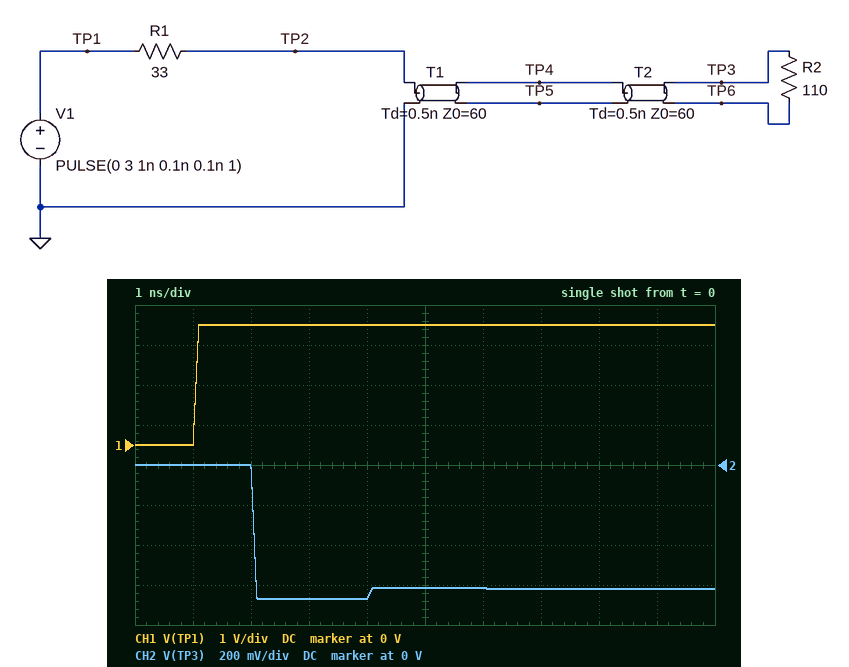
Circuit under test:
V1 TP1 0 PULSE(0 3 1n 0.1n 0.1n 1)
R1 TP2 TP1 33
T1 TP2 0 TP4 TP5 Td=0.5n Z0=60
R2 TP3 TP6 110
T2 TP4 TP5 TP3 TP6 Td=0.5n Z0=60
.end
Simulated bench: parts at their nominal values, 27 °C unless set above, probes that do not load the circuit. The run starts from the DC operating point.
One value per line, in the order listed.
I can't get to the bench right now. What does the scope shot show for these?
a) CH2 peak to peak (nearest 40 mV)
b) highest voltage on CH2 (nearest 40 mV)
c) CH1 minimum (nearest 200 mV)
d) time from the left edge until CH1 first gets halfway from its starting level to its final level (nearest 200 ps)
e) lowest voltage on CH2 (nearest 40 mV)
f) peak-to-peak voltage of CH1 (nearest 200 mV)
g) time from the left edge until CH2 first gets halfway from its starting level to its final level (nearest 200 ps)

680 mV
0 V
0 V
1.0 ns
-680 mV
3.0 V
2.0 ns
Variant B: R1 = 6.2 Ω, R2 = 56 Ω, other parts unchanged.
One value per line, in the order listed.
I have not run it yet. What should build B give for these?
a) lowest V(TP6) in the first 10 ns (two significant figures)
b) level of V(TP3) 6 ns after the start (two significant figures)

-4.1 V
-1.4 V
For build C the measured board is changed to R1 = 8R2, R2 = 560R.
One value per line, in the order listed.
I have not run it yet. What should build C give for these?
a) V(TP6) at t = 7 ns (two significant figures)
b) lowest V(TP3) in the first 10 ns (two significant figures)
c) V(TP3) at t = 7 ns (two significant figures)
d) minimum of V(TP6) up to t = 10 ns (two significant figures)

-3.8 V
-250 mV
-190 mV
-5.0 V
